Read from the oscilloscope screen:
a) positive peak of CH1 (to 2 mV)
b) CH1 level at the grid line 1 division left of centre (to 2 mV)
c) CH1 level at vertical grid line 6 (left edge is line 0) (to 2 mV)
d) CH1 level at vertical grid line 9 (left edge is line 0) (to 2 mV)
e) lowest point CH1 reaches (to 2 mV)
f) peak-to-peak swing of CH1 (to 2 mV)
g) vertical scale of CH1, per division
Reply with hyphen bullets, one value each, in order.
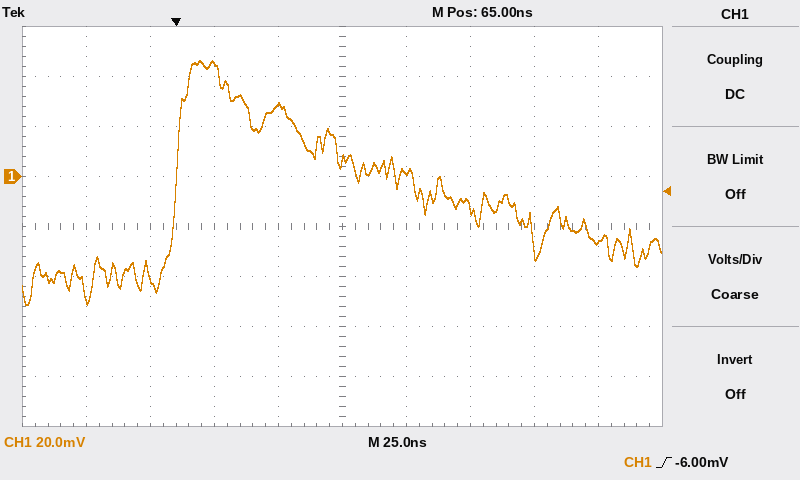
- 46 mV
- 28 mV
- 2 mV
- -26 mV
- -52 mV
- 98 mV
- 20 mV
